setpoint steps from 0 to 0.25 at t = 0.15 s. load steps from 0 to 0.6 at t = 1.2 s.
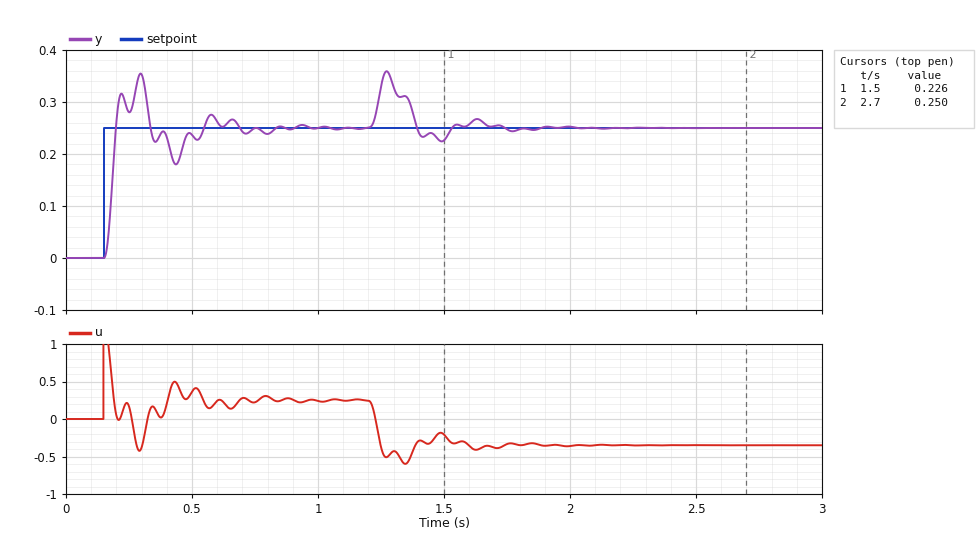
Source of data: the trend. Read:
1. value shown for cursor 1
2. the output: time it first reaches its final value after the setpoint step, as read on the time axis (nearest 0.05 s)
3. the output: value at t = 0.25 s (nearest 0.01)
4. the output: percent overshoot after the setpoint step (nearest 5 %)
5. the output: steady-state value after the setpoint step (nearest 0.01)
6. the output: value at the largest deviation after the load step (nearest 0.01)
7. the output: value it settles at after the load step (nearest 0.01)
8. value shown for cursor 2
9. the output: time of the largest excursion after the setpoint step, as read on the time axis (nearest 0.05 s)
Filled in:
0.226
0.20 s
0.28
40 %
0.25
0.36
0.25
0.250
0.30 s
